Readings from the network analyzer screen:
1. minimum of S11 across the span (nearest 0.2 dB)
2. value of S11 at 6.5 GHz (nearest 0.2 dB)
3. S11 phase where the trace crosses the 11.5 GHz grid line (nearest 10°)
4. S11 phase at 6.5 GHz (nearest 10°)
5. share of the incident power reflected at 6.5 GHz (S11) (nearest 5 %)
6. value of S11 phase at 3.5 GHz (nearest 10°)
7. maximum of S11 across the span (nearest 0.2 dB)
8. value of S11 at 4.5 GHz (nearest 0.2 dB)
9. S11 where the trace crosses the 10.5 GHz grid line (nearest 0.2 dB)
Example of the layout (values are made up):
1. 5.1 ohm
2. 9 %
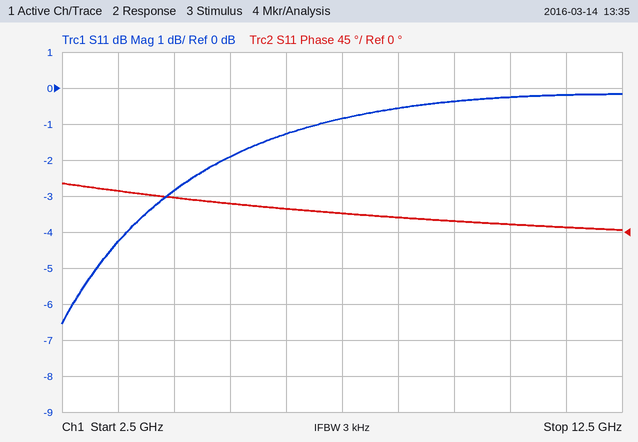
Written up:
1. -6.6 dB
2. -1.2 dB
3. 10°
4. 30°
5. 75 %
6. 50°
7. -0.2 dB
8. -2.8 dB
9. -0.2 dB
